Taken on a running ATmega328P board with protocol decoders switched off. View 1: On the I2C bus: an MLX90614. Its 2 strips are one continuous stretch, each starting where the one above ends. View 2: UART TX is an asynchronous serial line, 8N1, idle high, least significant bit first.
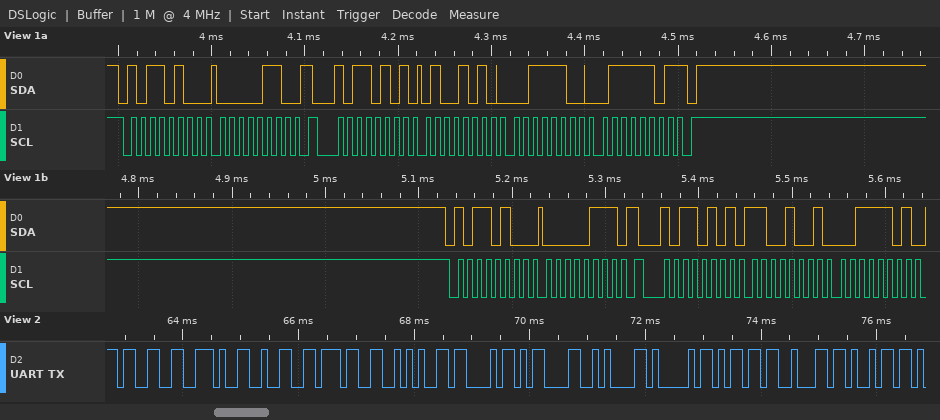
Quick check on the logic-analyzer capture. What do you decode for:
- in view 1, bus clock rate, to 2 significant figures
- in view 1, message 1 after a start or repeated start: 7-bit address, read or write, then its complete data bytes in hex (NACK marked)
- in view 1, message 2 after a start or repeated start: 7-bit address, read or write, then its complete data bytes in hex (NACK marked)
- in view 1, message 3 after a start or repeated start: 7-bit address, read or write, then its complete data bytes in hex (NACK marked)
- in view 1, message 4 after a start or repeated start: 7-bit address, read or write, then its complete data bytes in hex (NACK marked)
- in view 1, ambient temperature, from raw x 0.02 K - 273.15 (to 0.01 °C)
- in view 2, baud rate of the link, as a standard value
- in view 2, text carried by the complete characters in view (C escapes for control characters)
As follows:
100 kHz
0x5A write: 06
0x5A read: 4A 3C 7D NACK
0x5A write: 07
0x5A read: C9 3D
35.53 °C
9600 baud
"3.27*C\r\nAmbi"
